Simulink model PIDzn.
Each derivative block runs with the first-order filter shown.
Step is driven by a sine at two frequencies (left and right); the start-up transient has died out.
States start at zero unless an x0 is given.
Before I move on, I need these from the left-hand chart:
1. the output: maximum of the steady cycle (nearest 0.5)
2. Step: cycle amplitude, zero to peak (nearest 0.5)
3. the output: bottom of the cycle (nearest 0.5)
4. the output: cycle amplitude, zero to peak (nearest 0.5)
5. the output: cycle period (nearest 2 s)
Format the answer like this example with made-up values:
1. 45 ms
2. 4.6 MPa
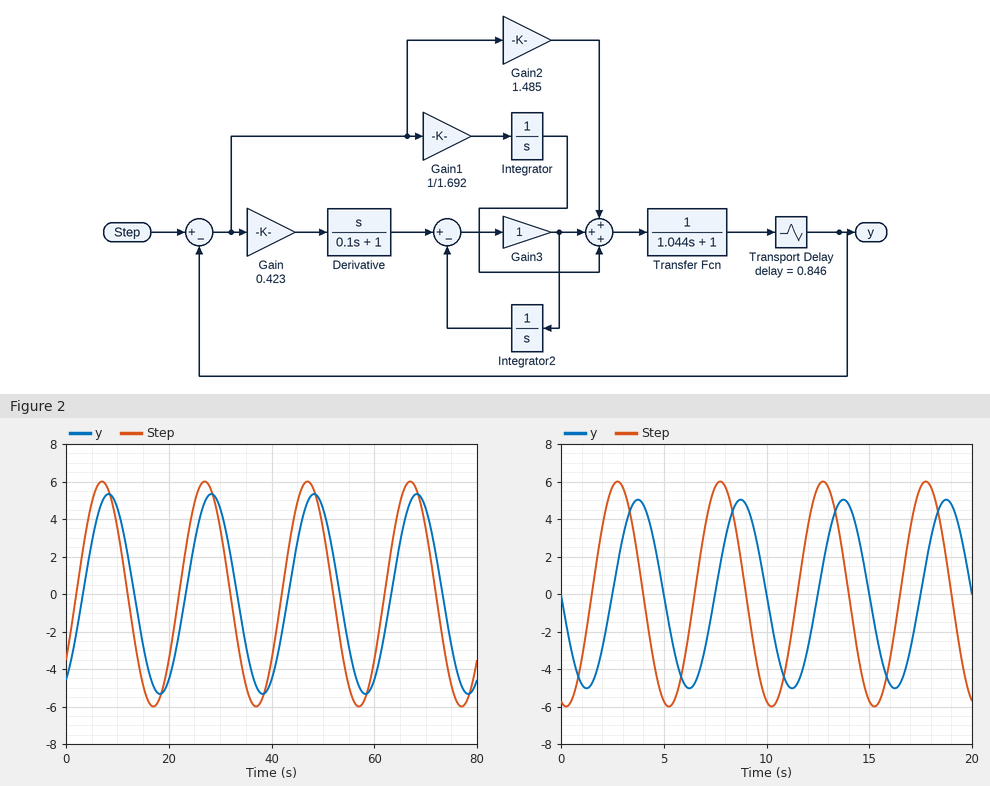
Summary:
1. 5.5
2. 6.0
3. -5.5
4. 5.5
5. 20 s
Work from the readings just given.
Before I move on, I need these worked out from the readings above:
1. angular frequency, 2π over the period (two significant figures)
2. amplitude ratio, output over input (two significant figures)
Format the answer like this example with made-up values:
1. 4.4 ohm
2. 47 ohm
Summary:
1. 0.31 rad/s
2. 0.92
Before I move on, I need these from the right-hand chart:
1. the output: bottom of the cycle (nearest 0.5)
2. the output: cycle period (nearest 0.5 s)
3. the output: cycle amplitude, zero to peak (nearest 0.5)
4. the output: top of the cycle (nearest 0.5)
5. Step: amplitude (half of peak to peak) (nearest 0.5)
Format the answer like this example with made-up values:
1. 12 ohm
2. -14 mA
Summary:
1. -5.0
2. 5.0 s
3. 5.0
4. 5.0
5. 6.0
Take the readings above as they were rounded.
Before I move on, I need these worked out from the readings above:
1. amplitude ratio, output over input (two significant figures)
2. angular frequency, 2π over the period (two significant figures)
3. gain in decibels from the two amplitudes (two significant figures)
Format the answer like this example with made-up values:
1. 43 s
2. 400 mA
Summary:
1. 0.83
2. 1.3 rad/s
3. -1.6 dB
